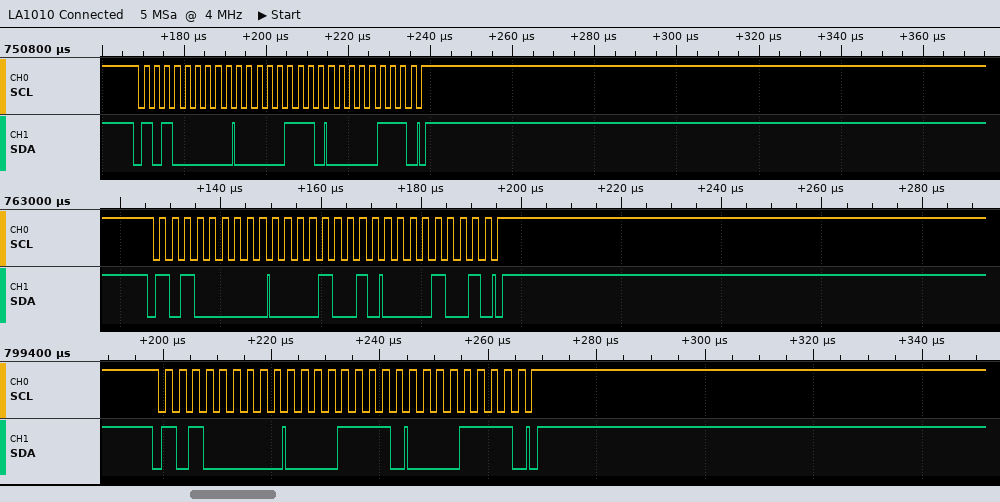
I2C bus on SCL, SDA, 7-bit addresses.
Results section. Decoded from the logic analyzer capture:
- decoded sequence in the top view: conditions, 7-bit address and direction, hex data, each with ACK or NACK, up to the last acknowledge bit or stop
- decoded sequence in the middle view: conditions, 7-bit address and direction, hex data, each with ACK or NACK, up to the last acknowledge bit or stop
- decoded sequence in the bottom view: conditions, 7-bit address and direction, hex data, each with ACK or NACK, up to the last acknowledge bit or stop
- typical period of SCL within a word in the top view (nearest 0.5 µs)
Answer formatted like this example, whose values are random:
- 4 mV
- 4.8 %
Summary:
- start, address 50 write ACK, 07 ACK, 07 ACK, stop
- start, address 50 write ACK, 09 ACK, 09 ACK, stop
- start, address 50 write ACK, 0F ACK, 0F ACK, stop
- 2.5 µs
